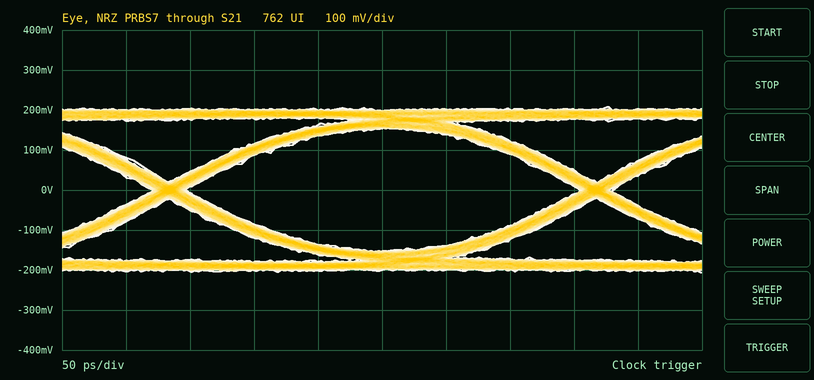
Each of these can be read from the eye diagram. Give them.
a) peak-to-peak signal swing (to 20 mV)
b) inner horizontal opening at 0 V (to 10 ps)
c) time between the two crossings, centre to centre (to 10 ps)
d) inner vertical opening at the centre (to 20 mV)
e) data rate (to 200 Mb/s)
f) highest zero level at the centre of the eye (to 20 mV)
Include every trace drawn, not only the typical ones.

420 mV
310 ps
330 ps
300 mV
3.0 Gb/s
-160 mV
